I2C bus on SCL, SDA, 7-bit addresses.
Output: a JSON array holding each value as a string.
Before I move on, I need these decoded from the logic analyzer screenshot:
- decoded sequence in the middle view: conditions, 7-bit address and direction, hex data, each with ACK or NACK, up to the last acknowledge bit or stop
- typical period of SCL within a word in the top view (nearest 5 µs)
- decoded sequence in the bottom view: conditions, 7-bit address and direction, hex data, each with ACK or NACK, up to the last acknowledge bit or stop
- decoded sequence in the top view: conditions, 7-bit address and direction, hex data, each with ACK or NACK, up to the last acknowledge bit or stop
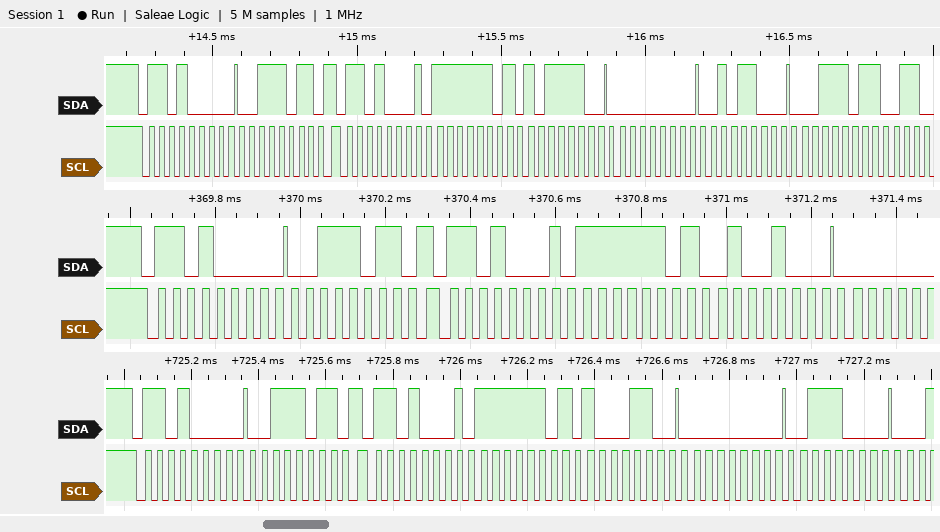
["start, address 68 write ACK, 3B ACK, repeated start, address 68 read ACK, FD ACK, 48 ACK", "35 µs", "start, address 68 write ACK, 3B ACK, repeated start, address 68 read ACK, FD ACK, 8C ACK, 00 ACK, 70 ACK", "start, address 68 write ACK, 3B ACK, repeated start, address 68 read ACK, FD ACK, BC ACK, 00 ACK, 58 ACK, 3B ACK"]
